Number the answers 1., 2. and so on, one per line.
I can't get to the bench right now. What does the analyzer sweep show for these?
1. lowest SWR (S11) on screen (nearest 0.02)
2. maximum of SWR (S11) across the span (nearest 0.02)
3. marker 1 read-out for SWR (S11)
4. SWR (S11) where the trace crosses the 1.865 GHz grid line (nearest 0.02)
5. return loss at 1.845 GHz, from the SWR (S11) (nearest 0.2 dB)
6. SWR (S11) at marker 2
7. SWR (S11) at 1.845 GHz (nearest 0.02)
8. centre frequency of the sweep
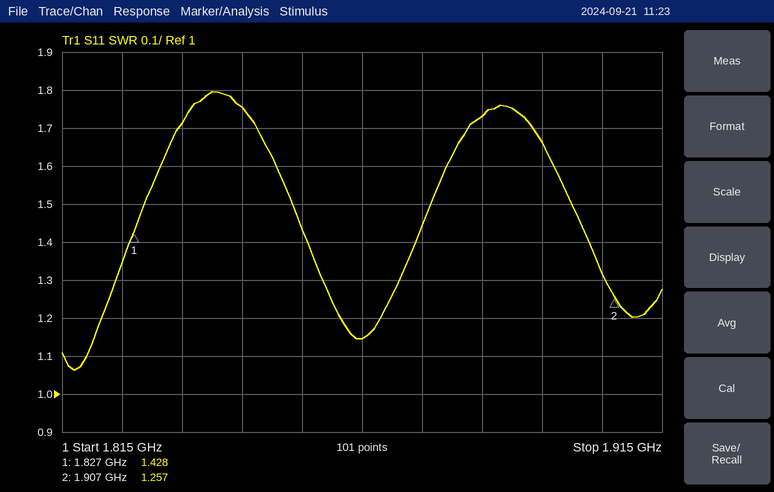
1. 1.06
2. 1.80
3. 1.428
4. 1.14
5. 11.2 dB
6. 1.257
7. 1.76
8. 1.865 GHz
